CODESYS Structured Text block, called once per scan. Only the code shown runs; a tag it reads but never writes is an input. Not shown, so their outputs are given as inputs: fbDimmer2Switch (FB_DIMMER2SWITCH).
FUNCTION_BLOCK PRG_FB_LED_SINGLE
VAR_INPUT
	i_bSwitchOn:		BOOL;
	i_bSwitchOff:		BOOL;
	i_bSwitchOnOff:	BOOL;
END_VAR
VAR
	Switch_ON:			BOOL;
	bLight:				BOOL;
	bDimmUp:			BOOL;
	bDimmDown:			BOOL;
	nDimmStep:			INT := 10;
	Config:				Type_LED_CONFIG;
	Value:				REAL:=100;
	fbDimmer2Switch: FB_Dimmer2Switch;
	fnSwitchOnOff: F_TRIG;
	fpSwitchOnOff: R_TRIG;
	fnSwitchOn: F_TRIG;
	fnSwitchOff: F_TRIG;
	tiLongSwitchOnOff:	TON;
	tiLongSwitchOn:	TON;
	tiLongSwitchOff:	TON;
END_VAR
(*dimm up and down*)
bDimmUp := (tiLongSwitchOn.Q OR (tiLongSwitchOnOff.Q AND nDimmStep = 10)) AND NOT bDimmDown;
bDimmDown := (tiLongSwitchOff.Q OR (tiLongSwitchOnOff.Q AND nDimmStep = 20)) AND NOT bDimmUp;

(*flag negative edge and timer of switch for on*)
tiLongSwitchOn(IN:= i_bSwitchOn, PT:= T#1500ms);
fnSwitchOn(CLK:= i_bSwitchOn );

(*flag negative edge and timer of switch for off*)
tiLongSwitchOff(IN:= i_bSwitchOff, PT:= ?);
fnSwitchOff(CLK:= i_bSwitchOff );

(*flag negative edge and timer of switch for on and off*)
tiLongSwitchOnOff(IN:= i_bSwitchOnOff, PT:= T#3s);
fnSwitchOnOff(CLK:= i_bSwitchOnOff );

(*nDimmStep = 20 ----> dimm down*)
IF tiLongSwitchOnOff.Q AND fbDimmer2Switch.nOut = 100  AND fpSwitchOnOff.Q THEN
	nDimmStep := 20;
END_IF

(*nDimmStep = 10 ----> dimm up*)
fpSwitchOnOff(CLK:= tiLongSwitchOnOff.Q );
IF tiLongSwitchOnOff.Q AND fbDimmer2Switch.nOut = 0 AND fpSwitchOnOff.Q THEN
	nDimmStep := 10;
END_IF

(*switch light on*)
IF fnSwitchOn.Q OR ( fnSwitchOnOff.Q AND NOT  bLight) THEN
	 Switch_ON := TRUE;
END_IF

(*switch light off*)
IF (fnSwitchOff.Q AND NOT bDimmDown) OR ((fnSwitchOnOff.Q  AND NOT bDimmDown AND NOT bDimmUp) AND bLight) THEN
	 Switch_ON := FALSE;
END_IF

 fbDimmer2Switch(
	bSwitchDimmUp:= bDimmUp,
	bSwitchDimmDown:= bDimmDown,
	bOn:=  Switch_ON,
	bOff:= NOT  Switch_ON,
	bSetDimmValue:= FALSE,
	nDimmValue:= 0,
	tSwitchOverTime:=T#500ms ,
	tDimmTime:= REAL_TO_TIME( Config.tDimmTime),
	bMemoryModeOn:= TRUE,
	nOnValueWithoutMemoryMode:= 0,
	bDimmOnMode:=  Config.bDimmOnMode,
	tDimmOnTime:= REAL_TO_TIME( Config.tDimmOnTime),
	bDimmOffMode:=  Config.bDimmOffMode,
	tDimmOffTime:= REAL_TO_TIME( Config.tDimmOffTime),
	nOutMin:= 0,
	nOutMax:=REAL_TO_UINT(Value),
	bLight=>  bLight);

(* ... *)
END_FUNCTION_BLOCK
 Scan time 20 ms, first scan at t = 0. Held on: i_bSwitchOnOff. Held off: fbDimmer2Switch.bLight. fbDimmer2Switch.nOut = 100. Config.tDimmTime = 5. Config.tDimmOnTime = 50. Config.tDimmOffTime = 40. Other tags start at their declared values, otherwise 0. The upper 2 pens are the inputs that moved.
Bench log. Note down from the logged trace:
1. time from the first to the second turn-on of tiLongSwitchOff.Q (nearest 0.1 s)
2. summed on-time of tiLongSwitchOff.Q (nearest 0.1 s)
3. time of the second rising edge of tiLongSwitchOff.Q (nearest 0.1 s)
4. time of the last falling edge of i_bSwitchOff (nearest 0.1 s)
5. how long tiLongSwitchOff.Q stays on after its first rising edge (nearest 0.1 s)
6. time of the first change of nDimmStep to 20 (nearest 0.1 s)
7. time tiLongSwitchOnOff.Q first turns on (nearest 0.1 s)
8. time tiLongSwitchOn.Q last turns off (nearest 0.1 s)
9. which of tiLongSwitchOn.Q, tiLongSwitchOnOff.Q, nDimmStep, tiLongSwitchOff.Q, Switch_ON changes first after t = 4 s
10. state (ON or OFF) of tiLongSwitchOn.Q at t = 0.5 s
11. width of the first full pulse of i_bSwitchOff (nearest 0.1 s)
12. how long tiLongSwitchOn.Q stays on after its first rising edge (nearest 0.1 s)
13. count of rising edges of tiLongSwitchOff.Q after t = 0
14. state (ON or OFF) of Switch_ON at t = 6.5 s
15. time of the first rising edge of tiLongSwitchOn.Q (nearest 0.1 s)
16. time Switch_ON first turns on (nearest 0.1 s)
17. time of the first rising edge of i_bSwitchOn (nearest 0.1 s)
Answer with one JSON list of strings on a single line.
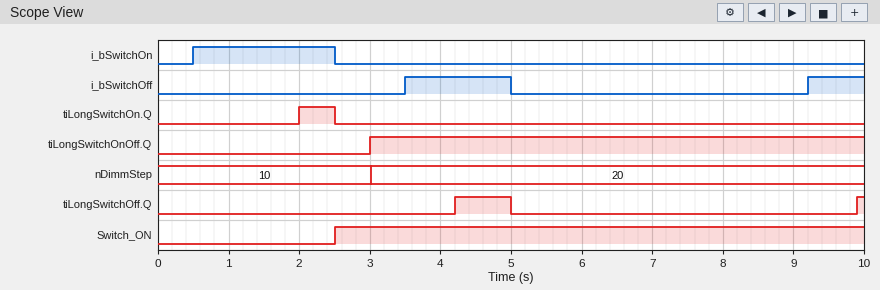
["5.7 s", "0.9 s", "9.9 s", "5.0 s", "0.8 s", "3.0 s", "3.0 s", "2.5 s", "tiLongSwitchOff.Q", "OFF", "1.5 s", "0.5 s", "2", "ON", "2.0 s", "2.5 s", "0.5 s"]
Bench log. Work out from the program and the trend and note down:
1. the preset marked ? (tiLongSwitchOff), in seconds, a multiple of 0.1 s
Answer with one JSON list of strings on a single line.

["0.7 s"]
